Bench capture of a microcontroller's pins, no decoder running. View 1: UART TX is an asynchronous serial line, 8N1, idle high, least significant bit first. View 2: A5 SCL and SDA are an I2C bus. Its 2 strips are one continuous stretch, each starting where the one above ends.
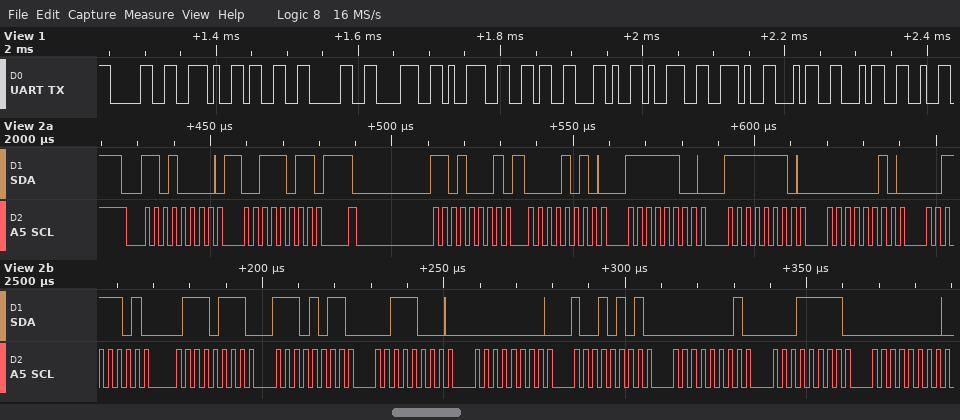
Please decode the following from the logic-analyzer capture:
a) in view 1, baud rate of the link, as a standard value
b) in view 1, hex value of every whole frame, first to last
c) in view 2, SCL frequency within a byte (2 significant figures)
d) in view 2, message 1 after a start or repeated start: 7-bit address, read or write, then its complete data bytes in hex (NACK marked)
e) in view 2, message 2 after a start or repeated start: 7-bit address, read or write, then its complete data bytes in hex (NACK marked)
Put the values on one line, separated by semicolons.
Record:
115200 baud; 30 2E 33 30 38 39 36 2C 39 2E 34 34; 400 kHz; 0x68 write: 3B; 0x68 read: 0A FC FE 02 3D 77 EB 38 00 95 01 1F 00
